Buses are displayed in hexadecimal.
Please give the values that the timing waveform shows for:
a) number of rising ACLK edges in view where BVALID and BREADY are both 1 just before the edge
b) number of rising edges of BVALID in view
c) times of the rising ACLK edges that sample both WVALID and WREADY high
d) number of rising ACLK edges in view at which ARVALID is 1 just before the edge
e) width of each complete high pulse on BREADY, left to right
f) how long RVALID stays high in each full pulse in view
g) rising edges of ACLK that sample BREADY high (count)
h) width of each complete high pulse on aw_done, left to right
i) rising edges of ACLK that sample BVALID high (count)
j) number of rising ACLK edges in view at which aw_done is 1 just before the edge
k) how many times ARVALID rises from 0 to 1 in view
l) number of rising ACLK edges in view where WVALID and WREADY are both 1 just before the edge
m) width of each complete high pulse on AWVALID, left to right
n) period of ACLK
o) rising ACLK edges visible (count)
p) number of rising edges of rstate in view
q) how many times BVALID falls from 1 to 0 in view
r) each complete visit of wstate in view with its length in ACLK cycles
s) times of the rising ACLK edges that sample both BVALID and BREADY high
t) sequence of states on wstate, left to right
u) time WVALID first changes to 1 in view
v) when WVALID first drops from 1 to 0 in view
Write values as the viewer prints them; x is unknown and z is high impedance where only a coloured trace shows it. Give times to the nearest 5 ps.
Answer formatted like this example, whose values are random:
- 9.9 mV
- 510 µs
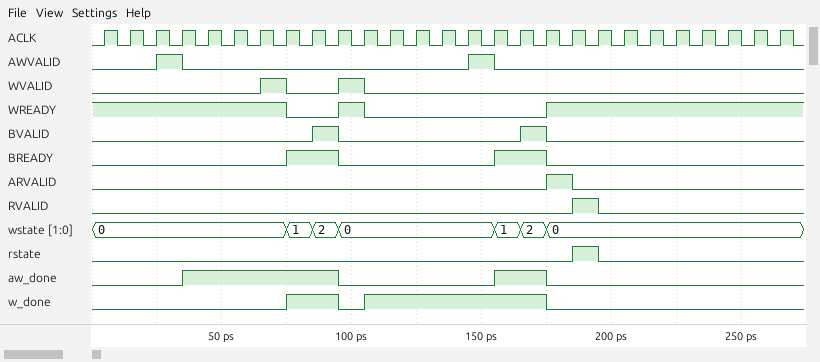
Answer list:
- 2
- 2
- 75 ps, 105 ps
- 1
- 20 ps, 20 ps
- 10 ps
- 4
- 60 ps, 20 ps
- 2
- 8
- 1
- 2
- 10 ps, 10 ps
- 10 ps
- 27
- 1
- 2
- 1: 1, 2: 1, 0: 6, 1: 1, 2: 1
- 95 ps, 175 ps
- 0, 1, 2, 0, 1, 2, 0
- 65 ps
- 75 ps
